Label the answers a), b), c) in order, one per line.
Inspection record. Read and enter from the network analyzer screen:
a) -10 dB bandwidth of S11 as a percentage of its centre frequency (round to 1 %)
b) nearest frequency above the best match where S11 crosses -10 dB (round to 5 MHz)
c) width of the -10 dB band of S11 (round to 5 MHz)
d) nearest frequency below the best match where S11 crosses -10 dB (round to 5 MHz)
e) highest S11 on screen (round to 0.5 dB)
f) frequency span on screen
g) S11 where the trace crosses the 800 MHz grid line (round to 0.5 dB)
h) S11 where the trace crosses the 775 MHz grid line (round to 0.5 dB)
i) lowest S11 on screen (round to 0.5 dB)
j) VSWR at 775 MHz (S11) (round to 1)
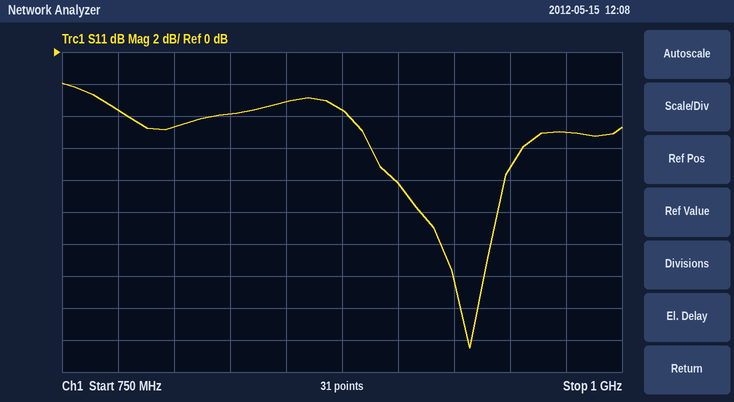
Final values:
a) 4 %
b) 945 MHz
c) 35 MHz
d) 910 MHz
e) -2.0 dB
f) 250 MHz
g) -4.5 dB
h) -3.5 dB
i) -18.5 dB
j) 5
